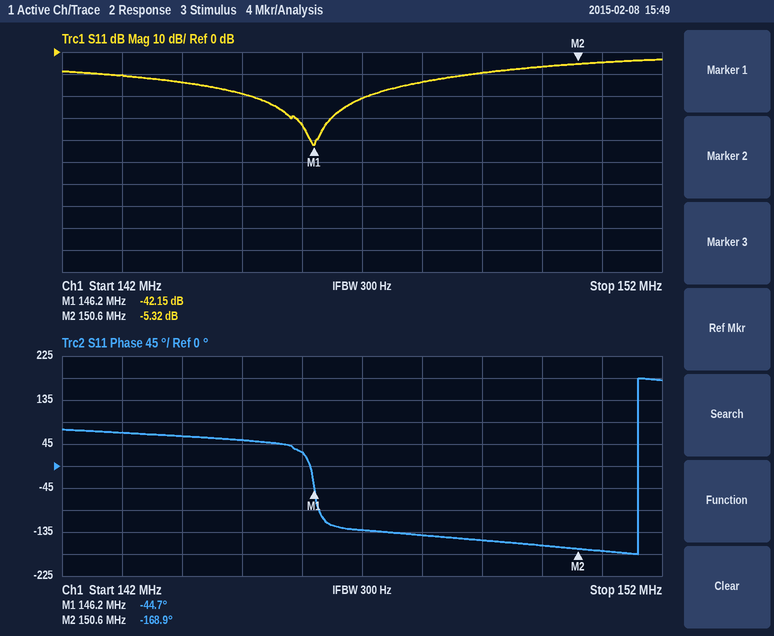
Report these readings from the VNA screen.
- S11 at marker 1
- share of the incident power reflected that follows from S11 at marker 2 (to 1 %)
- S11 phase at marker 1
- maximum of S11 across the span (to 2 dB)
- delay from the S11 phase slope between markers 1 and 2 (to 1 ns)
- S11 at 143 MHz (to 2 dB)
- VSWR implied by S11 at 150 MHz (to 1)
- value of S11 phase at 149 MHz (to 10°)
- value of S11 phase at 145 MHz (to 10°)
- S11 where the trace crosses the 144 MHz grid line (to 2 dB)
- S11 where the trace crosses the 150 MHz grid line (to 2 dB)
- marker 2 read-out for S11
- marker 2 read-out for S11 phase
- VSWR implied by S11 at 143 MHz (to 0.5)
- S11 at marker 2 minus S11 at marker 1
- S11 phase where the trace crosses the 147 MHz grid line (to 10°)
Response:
-42.15 dB
29 %
-44.7°
-4 dB
78 ns
-10 dB
3
-150°
50°
-14 dB
-6 dB
-5.32 dB
-168.9°
2.0
36.83 dB
-130°
